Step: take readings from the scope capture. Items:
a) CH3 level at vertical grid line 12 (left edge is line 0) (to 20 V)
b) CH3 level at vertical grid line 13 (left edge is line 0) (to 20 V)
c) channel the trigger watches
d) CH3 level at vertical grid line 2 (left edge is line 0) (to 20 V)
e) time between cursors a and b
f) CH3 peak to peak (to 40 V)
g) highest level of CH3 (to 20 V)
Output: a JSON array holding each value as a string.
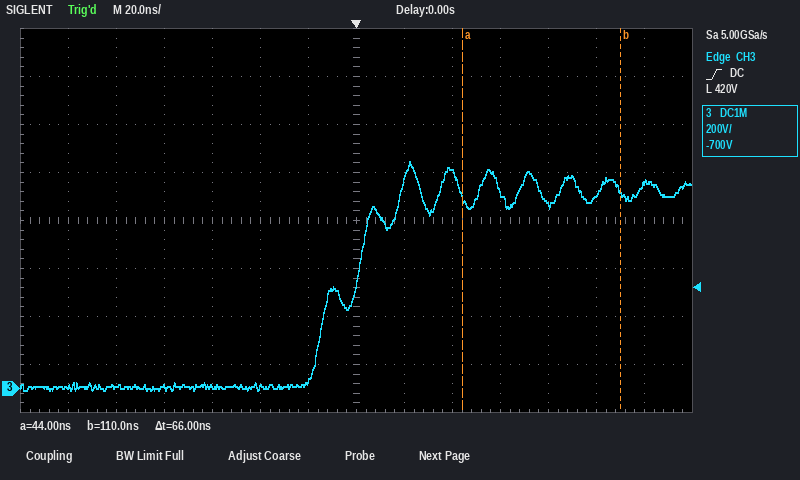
["800 V", "860 V", "CH3", "0 V", "66 ns", "960 V", "940 V"]
